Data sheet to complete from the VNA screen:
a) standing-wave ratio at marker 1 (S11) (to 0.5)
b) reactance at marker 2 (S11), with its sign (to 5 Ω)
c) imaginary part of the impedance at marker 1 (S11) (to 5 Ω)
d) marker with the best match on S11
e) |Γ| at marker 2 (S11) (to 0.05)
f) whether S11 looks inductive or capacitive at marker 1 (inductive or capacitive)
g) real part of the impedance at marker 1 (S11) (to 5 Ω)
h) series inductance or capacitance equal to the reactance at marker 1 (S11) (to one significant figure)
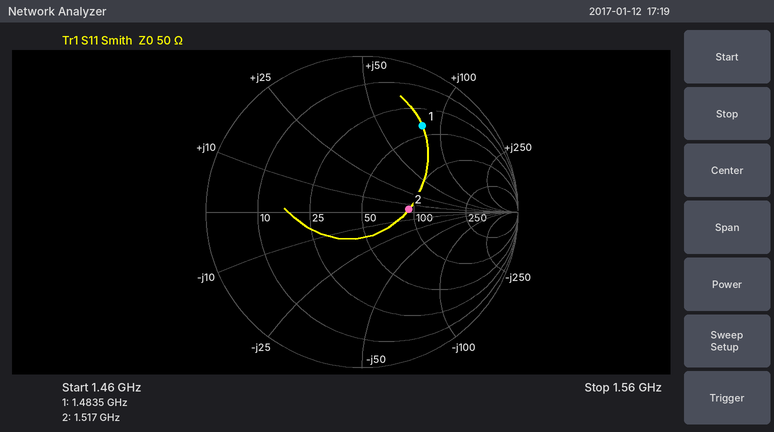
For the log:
5.0
+5 Ω
+80 Ω
marker 2
0.30
inductive
40 Ω
9 nH
